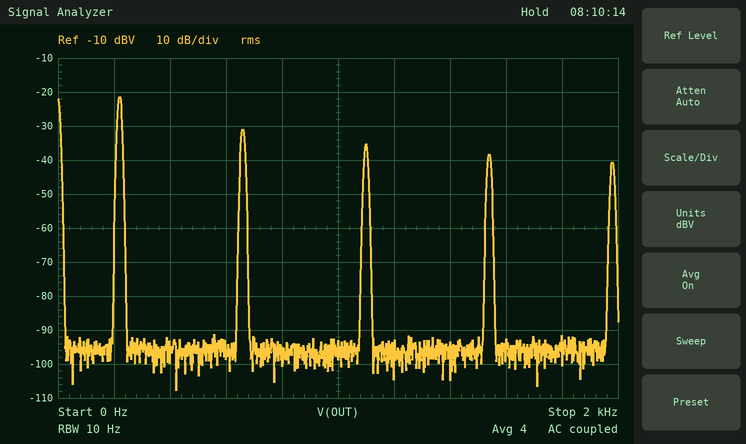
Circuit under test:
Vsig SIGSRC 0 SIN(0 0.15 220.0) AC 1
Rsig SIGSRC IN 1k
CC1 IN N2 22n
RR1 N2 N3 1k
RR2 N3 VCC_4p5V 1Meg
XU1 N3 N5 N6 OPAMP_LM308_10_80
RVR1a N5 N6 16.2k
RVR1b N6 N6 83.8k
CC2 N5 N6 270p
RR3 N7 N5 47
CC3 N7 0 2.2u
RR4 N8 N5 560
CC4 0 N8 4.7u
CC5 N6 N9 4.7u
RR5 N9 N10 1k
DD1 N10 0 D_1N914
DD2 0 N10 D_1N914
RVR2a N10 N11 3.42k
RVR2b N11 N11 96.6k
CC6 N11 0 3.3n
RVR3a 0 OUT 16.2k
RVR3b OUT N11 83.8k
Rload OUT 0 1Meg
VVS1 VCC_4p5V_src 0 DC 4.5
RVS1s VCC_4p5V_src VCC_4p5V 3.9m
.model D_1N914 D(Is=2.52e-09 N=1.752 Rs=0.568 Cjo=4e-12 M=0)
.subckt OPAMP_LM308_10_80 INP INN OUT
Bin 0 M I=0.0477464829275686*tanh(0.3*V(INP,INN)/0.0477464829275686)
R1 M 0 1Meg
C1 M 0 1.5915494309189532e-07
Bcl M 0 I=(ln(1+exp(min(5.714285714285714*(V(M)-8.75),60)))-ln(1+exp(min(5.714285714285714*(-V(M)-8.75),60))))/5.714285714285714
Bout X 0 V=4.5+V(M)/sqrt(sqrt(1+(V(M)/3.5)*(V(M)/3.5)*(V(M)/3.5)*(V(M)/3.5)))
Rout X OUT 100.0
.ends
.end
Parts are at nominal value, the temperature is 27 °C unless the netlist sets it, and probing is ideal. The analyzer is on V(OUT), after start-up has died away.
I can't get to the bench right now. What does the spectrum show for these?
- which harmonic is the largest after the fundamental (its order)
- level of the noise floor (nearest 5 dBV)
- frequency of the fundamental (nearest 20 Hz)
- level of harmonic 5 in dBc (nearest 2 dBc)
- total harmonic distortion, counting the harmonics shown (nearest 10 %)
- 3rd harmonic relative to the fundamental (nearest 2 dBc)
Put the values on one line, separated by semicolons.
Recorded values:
3; -95 dBV; 220 Hz; -14 dBc; 40 %; -10 dBc
